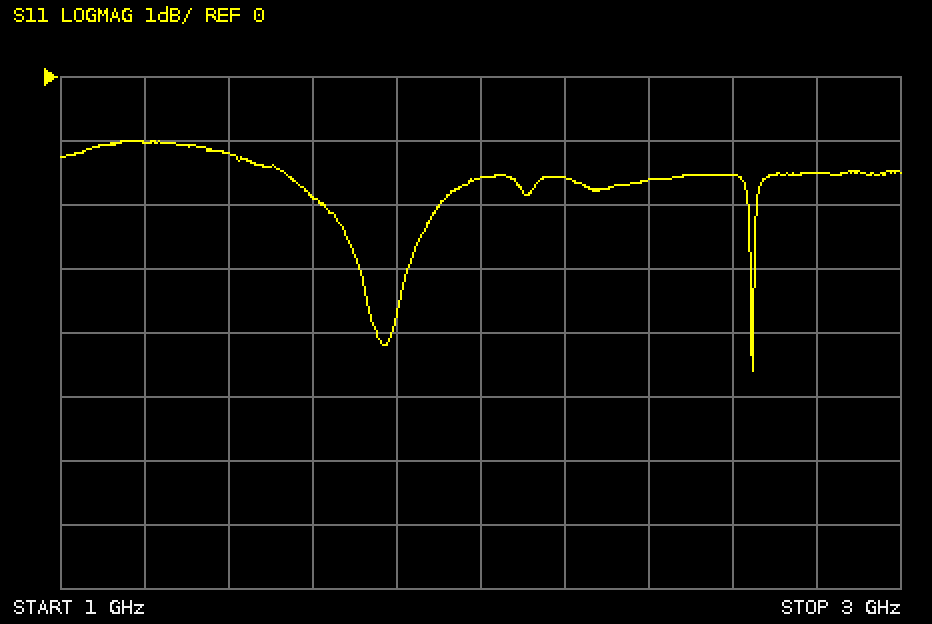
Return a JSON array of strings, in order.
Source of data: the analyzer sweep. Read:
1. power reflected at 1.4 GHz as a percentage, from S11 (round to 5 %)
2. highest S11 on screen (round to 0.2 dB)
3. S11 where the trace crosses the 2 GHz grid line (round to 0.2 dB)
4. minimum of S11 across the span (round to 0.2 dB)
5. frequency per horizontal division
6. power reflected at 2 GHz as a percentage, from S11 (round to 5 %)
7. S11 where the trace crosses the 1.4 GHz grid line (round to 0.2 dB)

["75 %", "-1.0 dB", "-1.6 dB", "-4.6 dB", "200 MHz", "70 %", "-1.2 dB"]
